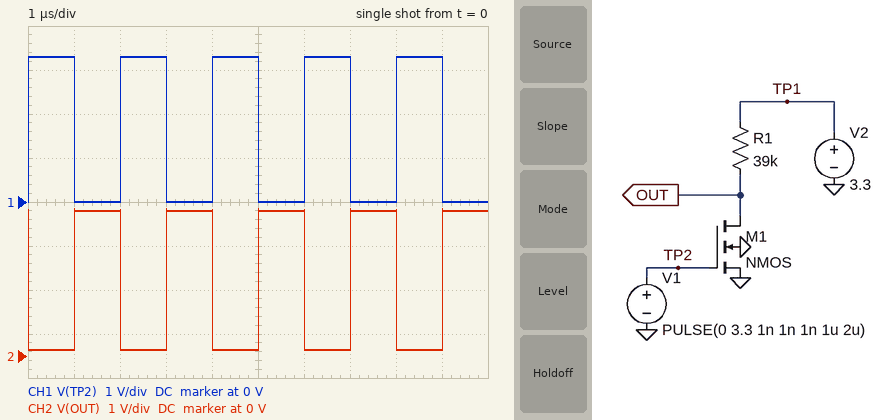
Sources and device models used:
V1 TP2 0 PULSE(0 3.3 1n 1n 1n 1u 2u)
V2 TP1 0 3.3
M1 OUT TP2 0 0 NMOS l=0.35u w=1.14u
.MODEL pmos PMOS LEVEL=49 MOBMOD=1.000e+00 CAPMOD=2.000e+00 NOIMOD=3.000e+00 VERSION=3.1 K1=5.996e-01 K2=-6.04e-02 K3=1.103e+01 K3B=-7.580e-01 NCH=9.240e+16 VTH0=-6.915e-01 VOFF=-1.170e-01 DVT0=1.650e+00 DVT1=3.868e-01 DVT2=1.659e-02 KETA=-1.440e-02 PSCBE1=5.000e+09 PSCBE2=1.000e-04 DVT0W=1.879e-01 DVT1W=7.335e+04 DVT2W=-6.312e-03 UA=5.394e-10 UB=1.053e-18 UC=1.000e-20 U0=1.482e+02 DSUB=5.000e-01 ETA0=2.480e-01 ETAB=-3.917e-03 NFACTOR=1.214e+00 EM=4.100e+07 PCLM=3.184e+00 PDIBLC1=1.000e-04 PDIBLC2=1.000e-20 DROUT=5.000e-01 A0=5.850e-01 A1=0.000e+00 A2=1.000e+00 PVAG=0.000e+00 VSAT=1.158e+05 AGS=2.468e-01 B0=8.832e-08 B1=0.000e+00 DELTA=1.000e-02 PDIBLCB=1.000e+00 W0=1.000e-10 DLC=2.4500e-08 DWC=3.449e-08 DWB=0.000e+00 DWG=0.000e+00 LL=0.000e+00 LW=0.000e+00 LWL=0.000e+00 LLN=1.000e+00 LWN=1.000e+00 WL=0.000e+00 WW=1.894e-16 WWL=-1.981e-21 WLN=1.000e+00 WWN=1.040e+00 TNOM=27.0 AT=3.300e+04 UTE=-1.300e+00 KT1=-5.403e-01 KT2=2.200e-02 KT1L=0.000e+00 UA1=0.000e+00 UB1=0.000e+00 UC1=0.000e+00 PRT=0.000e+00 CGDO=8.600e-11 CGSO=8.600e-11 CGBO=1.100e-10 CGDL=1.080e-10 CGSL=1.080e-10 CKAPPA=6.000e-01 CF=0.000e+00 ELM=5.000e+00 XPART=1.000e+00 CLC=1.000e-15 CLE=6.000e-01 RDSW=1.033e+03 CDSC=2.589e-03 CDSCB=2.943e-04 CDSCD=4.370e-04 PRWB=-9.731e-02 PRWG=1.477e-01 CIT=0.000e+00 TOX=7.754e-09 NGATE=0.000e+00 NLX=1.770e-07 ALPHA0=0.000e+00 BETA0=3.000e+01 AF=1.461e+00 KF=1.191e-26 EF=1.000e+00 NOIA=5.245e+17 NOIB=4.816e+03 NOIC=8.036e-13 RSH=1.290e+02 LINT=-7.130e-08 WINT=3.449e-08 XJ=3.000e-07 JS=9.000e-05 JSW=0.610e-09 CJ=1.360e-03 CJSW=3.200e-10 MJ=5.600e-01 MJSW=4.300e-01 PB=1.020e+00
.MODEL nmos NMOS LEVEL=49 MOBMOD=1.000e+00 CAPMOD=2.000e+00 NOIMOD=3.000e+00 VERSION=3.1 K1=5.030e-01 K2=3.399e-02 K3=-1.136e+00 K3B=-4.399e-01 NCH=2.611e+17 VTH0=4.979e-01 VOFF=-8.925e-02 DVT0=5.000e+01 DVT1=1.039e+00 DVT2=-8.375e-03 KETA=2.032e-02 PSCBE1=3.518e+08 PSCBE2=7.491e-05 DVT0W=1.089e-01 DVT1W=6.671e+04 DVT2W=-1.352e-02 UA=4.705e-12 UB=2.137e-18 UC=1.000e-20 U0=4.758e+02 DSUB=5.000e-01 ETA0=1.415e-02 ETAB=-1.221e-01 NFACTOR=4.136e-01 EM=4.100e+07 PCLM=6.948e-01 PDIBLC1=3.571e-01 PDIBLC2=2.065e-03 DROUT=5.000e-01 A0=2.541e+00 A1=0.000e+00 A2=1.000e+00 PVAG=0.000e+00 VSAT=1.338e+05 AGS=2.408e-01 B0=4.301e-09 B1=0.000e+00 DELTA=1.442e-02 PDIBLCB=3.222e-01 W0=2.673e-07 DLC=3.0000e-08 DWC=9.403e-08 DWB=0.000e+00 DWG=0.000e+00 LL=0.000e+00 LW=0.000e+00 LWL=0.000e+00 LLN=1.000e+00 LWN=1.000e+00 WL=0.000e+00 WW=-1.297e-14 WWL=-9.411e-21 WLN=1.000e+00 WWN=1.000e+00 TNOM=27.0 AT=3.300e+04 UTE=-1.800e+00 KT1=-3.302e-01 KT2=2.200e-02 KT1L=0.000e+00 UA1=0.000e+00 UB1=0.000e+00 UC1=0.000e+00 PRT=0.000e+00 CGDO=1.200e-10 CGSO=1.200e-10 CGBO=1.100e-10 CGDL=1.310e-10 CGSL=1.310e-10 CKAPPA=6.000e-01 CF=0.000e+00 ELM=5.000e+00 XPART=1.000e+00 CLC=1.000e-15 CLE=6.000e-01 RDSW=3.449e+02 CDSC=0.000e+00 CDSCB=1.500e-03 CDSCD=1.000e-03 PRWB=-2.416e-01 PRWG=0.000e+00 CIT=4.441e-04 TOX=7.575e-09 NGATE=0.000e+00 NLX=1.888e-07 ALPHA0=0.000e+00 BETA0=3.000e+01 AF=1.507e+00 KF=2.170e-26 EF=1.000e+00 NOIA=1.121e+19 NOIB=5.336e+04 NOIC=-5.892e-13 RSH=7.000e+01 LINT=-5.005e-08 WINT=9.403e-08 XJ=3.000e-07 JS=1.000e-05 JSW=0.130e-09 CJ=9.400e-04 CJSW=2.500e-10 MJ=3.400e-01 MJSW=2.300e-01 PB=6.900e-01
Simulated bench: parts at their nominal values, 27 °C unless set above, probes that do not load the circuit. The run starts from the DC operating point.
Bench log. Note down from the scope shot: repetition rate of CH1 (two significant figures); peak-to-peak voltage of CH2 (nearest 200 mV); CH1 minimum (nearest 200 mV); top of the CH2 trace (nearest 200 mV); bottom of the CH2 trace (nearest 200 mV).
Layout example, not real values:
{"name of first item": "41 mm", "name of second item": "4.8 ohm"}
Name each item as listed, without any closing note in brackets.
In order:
{"repetition rate of CH1": "500 kHz", "peak-to-peak voltage of CH2": "3.2 V", "CH1 minimum": "0 V", "top of the CH2 trace": "3.4 V", "bottom of the CH2 trace": "200 mV"}
